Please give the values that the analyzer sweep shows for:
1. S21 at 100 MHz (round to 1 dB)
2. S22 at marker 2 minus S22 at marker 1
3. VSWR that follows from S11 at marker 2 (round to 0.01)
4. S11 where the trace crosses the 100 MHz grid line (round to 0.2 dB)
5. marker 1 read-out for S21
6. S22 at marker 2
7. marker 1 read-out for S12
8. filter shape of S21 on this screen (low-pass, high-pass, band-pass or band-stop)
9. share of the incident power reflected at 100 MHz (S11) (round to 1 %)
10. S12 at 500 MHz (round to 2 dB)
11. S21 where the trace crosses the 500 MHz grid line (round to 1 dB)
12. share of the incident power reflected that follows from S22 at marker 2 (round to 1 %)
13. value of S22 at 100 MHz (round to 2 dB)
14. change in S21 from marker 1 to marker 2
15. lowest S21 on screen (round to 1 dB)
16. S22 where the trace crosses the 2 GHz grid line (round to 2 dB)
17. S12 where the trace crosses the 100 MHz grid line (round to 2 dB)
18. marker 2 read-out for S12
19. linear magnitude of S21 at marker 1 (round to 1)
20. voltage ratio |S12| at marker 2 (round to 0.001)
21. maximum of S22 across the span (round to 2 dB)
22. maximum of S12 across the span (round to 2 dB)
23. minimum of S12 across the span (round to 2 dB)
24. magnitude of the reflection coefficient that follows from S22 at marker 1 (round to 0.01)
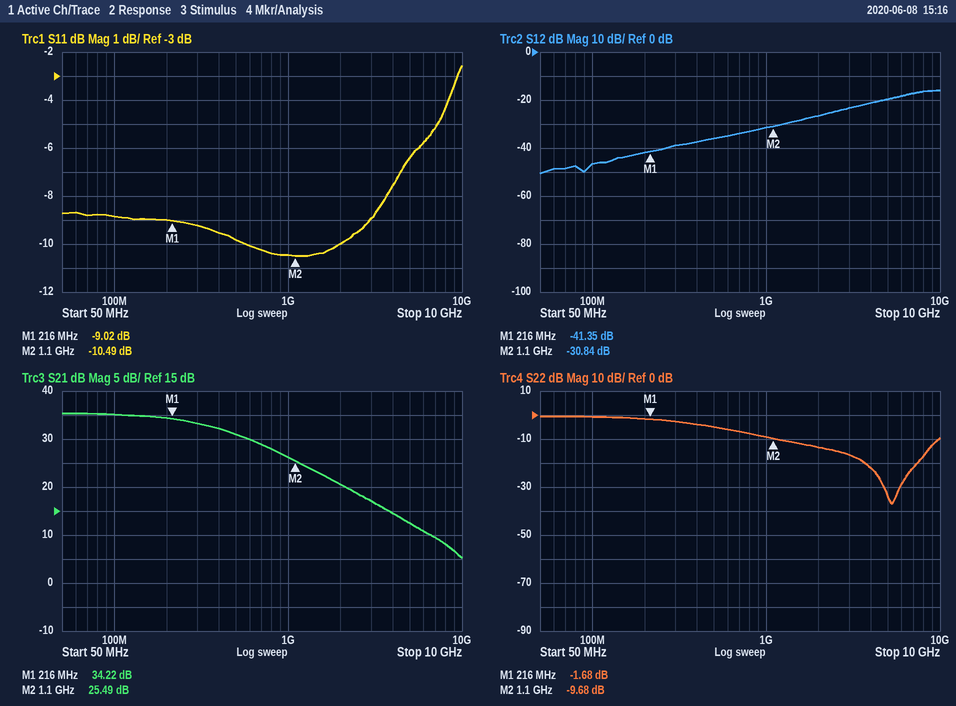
35 dB
-8.00 dB
1.85
-8.8 dB
34.22 dB
-9.68 dB
-41.35 dB
low-pass
13 %
-36 dB
31 dB
11 %
0 dB
-8.73 dB
5 dB
-14 dB
-46 dB
-30.84 dB
51
0.029
0 dB
-16 dB
-50 dB
0.82
